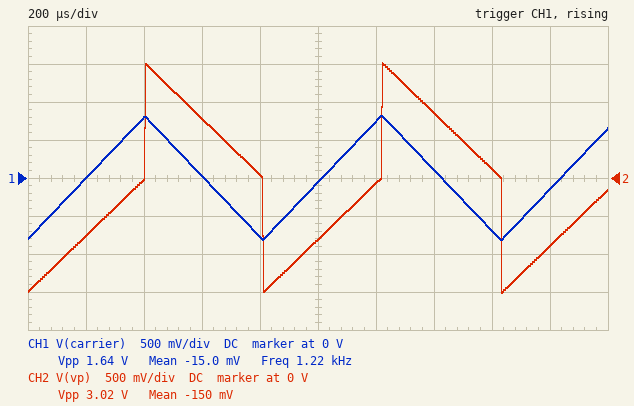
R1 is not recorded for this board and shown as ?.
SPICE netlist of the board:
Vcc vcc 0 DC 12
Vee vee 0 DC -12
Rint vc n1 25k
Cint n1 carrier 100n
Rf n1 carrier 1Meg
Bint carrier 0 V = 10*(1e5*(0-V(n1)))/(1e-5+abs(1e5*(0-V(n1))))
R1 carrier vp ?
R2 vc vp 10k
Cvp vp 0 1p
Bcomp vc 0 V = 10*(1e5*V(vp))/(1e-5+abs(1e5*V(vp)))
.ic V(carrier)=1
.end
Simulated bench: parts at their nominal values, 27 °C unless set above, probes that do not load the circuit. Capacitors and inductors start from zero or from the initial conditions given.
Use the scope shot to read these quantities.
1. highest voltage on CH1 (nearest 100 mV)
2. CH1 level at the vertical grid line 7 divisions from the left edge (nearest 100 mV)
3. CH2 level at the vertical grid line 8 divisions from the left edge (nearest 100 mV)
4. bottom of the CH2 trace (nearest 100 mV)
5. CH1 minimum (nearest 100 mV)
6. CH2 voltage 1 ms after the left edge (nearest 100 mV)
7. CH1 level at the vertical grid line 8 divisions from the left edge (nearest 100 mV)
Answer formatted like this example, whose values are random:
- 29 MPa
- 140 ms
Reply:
- 800 mV
- 100 mV
- 100 mV
- -1.5 V
- -800 mV
- -800 mV
- -700 mV
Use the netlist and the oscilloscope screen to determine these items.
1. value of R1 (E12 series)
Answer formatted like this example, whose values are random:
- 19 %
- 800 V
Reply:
- 820 Ω
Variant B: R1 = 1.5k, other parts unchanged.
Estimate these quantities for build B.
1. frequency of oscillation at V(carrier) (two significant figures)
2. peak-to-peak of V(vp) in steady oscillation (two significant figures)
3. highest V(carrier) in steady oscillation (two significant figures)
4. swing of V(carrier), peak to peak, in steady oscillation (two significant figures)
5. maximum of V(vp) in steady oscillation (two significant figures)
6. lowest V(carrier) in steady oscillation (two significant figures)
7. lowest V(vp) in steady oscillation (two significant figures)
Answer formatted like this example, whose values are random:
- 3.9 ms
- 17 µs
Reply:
- 670 Hz
- 5.2 V
- 1.5 V
- 3.0 V
- 2.6 V
- -1.5 V
- -2.6 V
